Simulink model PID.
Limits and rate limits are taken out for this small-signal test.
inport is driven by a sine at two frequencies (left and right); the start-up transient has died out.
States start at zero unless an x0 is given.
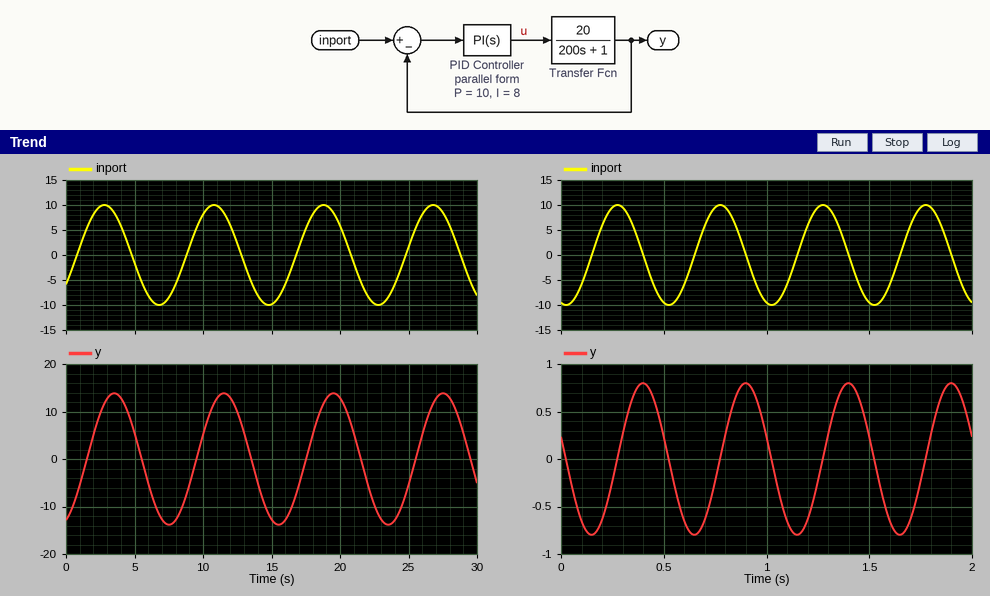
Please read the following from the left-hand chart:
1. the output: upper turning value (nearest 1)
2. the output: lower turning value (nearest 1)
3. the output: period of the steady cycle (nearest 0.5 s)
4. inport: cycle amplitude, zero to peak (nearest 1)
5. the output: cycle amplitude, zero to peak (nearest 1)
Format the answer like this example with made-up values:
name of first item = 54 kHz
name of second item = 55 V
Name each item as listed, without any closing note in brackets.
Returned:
the output: upper turning value = 14
the output: lower turning value = -14
the output: period of the steady cycle = 8.0 s
inport: cycle amplitude, zero to peak = 10
the output: cycle amplitude, zero to peak = 14
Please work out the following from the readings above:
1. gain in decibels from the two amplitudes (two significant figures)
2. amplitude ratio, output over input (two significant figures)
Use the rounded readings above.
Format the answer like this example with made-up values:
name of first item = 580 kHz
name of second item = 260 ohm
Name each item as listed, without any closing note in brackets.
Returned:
gain in decibels from the two amplitudes = 2.9 dB
amplitude ratio, output over input = 1.4
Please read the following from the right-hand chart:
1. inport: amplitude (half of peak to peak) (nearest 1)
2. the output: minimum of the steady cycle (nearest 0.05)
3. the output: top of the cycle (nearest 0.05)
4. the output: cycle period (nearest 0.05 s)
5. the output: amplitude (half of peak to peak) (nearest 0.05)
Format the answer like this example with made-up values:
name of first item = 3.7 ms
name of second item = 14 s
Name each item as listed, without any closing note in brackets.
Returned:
inport: amplitude (half of peak to peak) = 10
the output: minimum of the steady cycle = -0.80
the output: top of the cycle = 0.80
the output: cycle period = 0.50 s
the output: amplitude (half of peak to peak) = 0.80
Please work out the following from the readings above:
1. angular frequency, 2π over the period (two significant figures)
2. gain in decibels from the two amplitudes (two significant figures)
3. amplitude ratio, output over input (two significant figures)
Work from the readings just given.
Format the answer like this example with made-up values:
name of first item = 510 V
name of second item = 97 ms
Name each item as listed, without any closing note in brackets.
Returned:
angular frequency, 2π over the period = 13 rad/s
gain in decibels from the two amplitudes = -22 dB
amplitude ratio, output over input = 0.080
